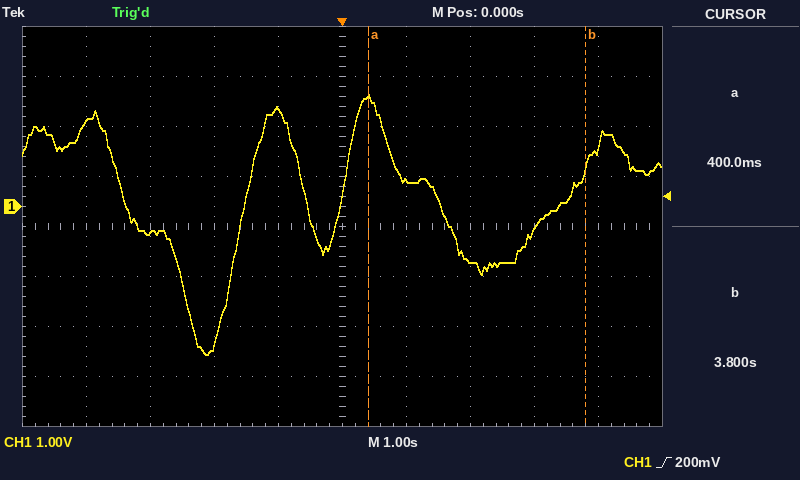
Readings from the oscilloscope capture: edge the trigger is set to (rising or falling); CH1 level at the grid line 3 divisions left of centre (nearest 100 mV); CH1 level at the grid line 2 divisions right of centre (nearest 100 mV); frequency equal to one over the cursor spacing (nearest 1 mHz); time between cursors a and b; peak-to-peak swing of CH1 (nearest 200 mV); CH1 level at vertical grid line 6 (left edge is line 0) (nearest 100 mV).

rising
-500 mV
-1.1 V
294 mHz
3.4 s
5.2 V
500 mV
